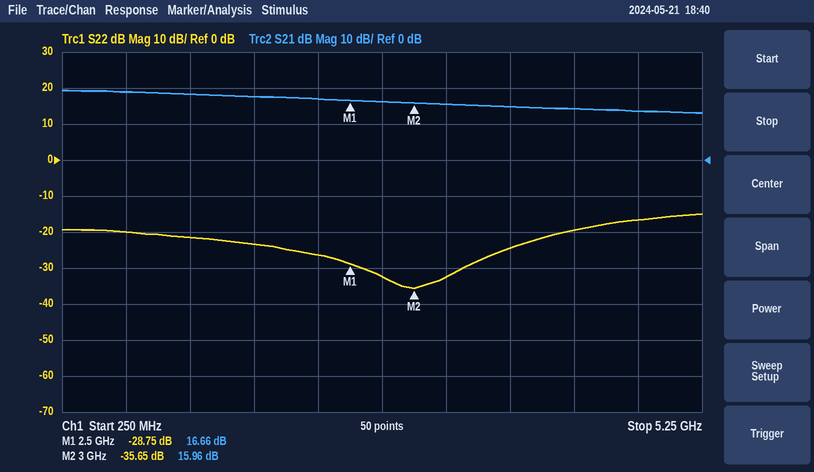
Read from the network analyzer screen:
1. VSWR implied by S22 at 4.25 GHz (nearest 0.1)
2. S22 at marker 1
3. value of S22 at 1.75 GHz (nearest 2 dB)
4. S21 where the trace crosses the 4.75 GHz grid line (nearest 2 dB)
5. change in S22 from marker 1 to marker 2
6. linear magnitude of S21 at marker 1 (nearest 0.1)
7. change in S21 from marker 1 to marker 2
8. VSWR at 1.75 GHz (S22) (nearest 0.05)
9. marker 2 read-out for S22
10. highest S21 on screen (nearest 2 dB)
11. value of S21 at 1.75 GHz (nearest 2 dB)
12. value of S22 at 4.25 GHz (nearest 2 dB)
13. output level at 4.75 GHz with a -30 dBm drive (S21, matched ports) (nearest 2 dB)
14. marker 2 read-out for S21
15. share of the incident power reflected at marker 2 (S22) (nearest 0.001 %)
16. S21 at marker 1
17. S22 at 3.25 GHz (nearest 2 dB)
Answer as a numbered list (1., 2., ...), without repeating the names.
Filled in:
1. 1.2
2. -28.75 dB
3. -24 dB
4. 14 dB
5. -6.90 dB
6. 6.8
7. -0.70 dB
8. 1.15
9. -35.65 dB
10. 20 dB
11. 18 dB
12. -20 dB
13. -16 dBm
14. 15.96 dB
15. 0.027 %
16. 16.66 dB
17. -32 dB
